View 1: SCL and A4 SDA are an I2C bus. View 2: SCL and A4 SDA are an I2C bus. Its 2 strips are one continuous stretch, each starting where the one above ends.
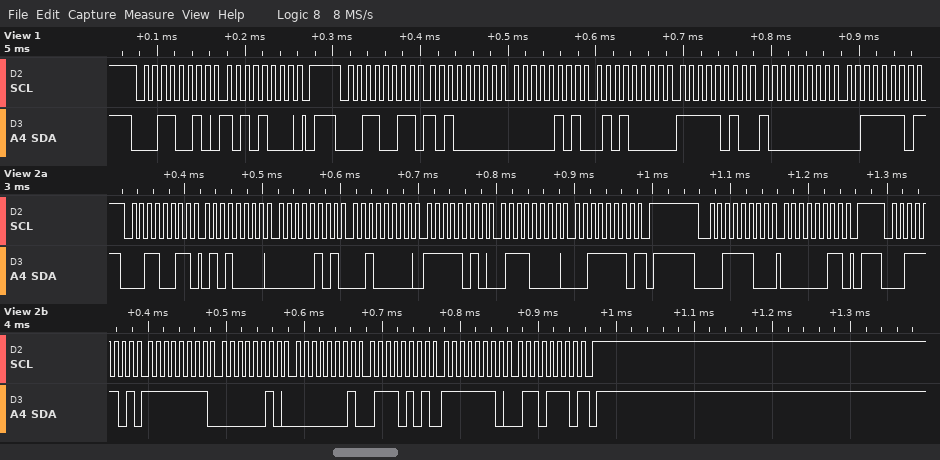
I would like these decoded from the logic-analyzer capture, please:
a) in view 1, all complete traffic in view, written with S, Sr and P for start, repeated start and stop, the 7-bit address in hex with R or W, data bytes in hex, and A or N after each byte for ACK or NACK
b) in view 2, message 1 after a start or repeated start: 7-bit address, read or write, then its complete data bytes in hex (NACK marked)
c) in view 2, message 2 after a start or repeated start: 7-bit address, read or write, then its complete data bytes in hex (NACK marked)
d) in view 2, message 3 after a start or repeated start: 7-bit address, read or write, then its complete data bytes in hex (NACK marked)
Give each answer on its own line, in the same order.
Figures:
S 19W A A8 A P S 19R A A0 A 05 A 50 A FA A 80 A 3E N
0x19 read: 50 05 20 FA 70 3E NACK
0x1E write: 03
0x1E read: FF 02 01 75 FE 6E NACK
